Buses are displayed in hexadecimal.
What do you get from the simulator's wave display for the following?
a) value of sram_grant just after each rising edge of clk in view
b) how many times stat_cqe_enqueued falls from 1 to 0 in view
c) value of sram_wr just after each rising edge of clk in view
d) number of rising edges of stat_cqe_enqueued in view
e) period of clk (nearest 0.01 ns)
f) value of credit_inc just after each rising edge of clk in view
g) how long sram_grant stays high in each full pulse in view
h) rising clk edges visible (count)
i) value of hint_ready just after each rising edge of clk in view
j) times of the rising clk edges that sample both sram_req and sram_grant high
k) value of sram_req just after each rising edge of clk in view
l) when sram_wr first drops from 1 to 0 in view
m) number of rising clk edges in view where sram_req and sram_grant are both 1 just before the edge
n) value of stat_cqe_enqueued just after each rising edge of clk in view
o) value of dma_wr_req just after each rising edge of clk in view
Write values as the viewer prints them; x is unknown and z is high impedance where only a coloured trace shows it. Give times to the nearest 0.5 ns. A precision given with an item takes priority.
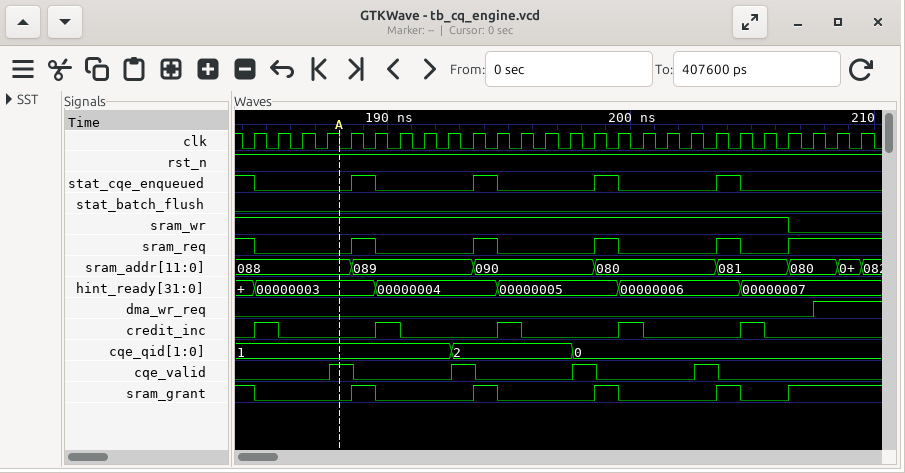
0 0 0 0 1 0 0 0 0 1 0 0 0 0 1 0 0 0 0 1 0 0 1 1 1 1
5
1 1 1 1 1 1 1 1 1 1 1 1 1 1 1 1 1 1 1 1 1 1 0 0 0 0
4
1 ns
1 0 0 0 0 1 0 0 0 0 1 0 0 0 0 1 0 0 0 0 1 0 0 0 0 0
1 ns, 1 ns, 1 ns, 1 ns
26
00000003, 00000003, 00000003, 00000003, 00000003, 00000004, 00000004, 00000004, 00000004, 00000004, 00000005, 00000005, 00000005, 00000005, 00000005, 00000006, 00000006, 00000006, 00000006, 00000006, 00000007, 00000007, 00000007, 00000007, 00000007, 00000007
184.5 ns, 189.5 ns, 194.5 ns, 199.5 ns, 204.5 ns, 207.5 ns, 208.5 ns, 209.5 ns
0 0 0 0 1 0 0 0 0 1 0 0 0 0 1 0 0 0 0 1 0 0 1 1 1 1
206.5 ns
8
0 0 0 0 1 0 0 0 0 1 0 0 0 0 1 0 0 0 0 1 0 0 0 0 0 0
0 0 0 0 0 0 0 0 0 0 0 0 0 0 0 0 0 0 0 0 0 0 0 1 1 1
